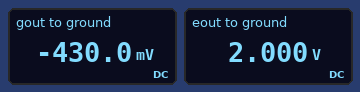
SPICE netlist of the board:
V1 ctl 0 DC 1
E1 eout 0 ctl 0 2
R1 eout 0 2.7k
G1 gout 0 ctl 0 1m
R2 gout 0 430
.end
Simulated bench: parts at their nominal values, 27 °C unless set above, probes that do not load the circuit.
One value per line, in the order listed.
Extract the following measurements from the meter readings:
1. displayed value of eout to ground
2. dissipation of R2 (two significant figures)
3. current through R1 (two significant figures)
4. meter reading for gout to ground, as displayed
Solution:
2.000 V
430 µW
740 µA
-430.0 mV
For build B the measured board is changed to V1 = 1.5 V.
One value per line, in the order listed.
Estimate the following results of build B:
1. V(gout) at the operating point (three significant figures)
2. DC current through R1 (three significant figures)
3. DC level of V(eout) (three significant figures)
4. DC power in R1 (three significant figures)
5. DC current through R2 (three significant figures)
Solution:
-645 mV
1.11 mA
3.00 V
3.33 mW
1.50 mA
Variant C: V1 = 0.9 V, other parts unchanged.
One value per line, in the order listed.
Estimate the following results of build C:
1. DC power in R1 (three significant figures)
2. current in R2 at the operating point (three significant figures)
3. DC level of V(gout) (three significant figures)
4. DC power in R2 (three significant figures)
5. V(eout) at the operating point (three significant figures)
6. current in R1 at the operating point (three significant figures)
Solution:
1.20 mW
900 µA
-387 mV
348 µW
1.80 V
667 µA
